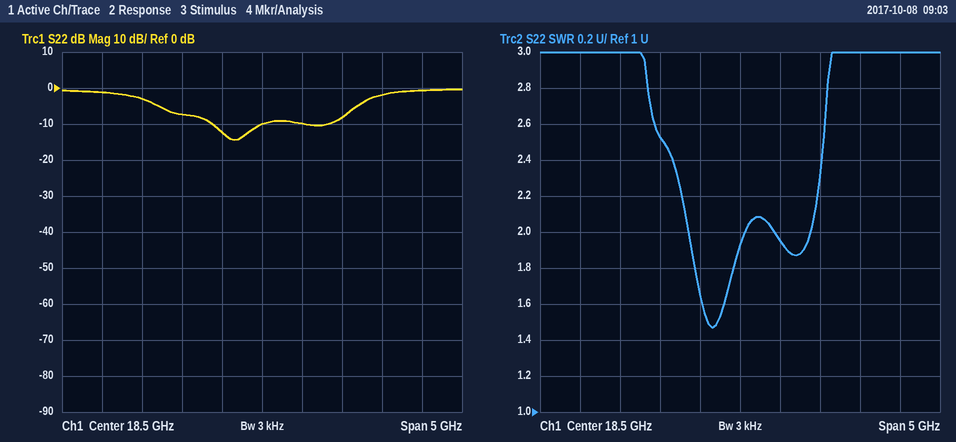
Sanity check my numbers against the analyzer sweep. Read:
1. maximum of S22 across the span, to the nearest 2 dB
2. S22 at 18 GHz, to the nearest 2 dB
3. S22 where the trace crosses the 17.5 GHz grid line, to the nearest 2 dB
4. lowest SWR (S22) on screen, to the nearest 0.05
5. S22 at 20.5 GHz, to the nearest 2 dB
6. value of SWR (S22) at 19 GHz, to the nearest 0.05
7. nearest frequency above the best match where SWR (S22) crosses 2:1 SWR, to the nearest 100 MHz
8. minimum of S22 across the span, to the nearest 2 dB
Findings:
0 dB
-12 dB
-8 dB
1.45
0 dB
1.95
18.6 GHz
-14 dB
